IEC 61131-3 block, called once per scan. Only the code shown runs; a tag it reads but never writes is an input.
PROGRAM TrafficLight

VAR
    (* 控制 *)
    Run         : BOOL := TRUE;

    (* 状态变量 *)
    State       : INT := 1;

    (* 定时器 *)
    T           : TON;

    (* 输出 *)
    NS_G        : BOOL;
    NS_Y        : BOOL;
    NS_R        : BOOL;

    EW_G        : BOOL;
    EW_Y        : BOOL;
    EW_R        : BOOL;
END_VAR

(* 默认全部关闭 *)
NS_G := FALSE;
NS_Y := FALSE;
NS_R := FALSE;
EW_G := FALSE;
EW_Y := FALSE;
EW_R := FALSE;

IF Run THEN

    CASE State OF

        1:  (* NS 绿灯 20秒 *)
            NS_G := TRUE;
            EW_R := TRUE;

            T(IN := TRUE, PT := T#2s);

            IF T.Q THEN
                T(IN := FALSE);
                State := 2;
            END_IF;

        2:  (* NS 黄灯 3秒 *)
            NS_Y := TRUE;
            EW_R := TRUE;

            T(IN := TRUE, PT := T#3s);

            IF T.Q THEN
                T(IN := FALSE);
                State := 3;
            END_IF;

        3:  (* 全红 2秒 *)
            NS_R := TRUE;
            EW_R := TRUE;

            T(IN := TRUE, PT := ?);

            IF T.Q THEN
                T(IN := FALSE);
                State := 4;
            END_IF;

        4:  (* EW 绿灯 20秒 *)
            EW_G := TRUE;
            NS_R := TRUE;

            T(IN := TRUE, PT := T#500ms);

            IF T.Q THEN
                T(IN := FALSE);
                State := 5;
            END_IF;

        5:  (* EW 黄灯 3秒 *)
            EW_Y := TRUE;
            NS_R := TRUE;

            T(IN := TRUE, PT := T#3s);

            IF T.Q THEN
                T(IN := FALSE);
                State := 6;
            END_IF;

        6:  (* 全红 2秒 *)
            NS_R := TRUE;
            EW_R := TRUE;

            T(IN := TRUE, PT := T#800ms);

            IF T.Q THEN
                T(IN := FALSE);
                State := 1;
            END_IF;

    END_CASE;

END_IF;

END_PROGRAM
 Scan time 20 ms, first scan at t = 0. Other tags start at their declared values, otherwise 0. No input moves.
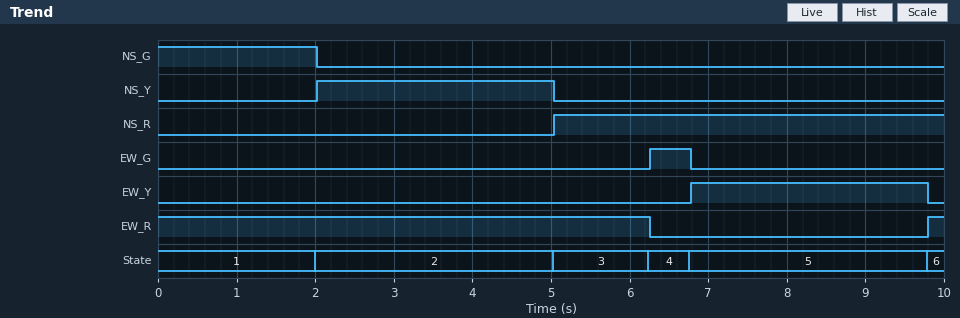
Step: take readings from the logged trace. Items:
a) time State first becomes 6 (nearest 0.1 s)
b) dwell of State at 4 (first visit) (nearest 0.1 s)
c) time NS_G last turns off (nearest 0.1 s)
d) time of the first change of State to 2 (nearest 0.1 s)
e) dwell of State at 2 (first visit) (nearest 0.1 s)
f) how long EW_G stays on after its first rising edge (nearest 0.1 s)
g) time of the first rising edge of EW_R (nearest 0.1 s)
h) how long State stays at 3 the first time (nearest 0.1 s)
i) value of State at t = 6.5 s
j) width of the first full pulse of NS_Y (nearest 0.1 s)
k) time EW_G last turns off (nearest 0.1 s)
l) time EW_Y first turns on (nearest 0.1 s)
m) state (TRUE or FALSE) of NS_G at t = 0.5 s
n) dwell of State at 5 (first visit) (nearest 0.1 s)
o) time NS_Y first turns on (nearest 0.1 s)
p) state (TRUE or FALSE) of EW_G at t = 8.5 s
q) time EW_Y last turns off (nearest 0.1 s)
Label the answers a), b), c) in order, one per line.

a) 9.8 s
b) 0.5 s
c) 2.0 s
d) 2.0 s
e) 3.0 s
f) 0.5 s
g) 9.8 s
h) 1.2 s
i) 4
j) 3.0 s
k) 6.8 s
l) 6.8 s
m) TRUE
n) 3.0 s
o) 2.0 s
p) FALSE
q) 9.8 s
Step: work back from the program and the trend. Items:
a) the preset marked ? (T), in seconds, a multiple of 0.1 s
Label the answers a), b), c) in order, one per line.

a) 1.2 s
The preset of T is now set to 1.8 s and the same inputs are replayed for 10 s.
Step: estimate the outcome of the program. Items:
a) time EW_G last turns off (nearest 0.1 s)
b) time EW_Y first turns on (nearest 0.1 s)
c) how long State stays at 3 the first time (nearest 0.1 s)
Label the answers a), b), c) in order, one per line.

a) 7.4 s
b) 7.4 s
c) 1.8 s
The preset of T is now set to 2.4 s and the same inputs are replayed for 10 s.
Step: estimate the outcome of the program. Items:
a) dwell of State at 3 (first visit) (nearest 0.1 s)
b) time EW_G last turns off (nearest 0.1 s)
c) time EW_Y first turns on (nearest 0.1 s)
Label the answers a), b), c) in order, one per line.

a) 2.4 s
b) 8.0 s
c) 8.0 s
